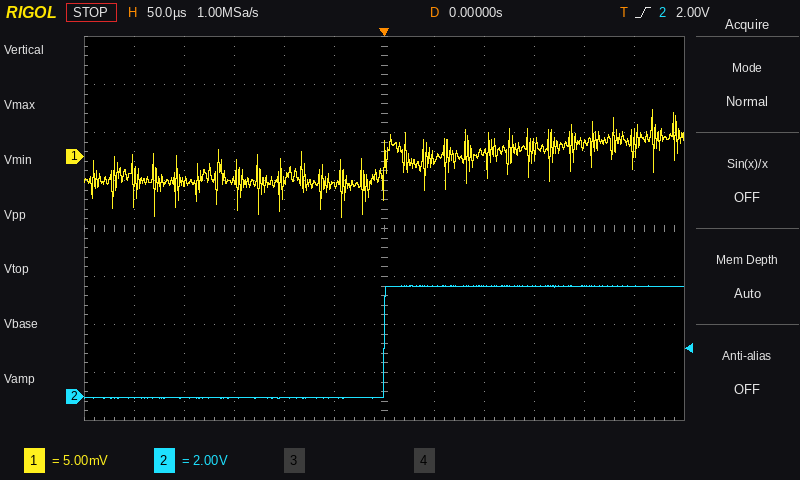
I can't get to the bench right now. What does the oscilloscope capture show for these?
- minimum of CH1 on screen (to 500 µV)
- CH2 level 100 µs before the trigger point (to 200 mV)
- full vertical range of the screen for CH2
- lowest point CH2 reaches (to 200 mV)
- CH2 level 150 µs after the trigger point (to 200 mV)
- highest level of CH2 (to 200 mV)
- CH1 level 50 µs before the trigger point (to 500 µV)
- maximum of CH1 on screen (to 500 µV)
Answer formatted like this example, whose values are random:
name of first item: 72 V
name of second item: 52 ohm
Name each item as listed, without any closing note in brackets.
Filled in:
minimum of CH1 on screen: -6.5 mV
CH2 level 100 µs before the trigger point: 0.0 V
full vertical range of the screen for CH2: 16 V
lowest point CH2 reaches: 0.0 V
CH2 level 150 µs after the trigger point: 4.6 V
highest level of CH2: 4.6 V
CH1 level 50 µs before the trigger point: -3.0 mV
maximum of CH1 on screen: 5.0 mV
